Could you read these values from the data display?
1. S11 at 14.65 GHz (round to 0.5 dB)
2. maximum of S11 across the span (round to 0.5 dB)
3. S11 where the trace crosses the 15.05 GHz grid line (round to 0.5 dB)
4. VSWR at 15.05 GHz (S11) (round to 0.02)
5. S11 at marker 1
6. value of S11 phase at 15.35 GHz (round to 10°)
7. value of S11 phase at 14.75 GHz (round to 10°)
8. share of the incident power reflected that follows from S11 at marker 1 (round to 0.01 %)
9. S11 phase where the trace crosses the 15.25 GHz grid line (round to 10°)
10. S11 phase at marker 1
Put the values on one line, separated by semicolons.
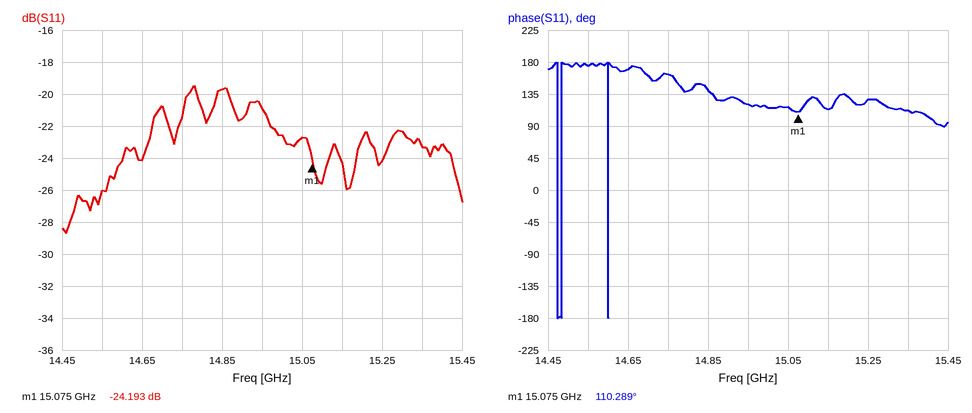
-24.0 dB; -19.5 dB; -22.5 dB; 1.16; -24.193 dB; 110°; 160°; 0.38 %; 130°; 110.289°
